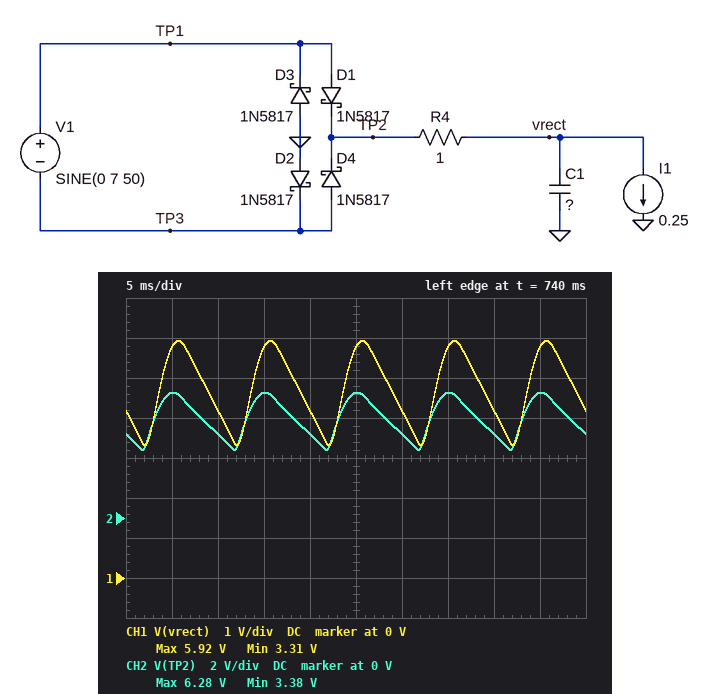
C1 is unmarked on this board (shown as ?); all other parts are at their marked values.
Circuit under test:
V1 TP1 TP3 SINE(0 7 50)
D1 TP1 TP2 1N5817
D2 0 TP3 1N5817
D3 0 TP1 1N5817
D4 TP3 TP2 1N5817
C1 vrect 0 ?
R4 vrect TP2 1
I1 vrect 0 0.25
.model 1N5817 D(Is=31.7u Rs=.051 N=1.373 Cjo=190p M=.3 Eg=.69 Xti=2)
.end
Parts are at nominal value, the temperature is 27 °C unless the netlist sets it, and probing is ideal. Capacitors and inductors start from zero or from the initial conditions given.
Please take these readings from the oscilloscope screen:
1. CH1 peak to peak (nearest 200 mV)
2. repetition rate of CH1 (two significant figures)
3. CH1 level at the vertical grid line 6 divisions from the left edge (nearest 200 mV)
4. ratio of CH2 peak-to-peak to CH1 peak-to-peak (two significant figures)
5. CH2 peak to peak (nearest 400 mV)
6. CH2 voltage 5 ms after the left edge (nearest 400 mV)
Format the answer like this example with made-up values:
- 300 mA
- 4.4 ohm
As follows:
- 2.6 V
- 100 Hz
- 4.2 V
- 1.1
- 2.8 V
- 6.4 V
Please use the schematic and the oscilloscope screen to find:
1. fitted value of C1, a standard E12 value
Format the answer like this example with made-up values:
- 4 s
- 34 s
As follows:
- 560 µF
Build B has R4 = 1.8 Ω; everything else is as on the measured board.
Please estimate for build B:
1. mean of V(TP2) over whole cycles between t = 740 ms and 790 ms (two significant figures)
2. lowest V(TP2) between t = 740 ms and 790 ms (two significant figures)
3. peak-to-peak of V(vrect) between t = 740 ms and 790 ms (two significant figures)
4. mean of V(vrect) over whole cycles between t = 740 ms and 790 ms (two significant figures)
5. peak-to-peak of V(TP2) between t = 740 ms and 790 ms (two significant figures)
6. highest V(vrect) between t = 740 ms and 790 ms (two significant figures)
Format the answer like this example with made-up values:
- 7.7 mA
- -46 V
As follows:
- 4.8 V
- 3.2 V
- 2.4 V
- 4.4 V
- 3.1 V
- 5.5 V
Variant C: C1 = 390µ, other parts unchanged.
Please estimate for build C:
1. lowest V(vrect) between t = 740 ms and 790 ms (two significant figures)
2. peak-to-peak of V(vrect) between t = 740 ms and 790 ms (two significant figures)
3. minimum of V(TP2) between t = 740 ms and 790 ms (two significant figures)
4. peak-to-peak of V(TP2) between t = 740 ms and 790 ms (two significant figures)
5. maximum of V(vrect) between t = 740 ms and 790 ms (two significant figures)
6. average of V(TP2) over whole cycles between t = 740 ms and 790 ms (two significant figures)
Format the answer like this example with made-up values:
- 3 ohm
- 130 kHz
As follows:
- 2.5 V
- 3.5 V
- 2.6 V
- 3.7 V
- 6.0 V
- 4.7 V
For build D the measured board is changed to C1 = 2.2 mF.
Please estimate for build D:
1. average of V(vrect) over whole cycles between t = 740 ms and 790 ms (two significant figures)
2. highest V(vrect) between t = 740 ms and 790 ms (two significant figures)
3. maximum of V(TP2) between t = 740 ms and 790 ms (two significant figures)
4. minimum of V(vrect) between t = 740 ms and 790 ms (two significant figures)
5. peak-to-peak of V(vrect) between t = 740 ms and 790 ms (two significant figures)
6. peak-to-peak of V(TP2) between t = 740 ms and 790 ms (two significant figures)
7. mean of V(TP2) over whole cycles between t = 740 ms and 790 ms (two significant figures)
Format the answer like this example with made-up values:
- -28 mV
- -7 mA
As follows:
- 5.1 V
- 5.5 V
- 6.2 V
- 4.8 V
- 720 mV
- 1.4 V
- 5.4 V
